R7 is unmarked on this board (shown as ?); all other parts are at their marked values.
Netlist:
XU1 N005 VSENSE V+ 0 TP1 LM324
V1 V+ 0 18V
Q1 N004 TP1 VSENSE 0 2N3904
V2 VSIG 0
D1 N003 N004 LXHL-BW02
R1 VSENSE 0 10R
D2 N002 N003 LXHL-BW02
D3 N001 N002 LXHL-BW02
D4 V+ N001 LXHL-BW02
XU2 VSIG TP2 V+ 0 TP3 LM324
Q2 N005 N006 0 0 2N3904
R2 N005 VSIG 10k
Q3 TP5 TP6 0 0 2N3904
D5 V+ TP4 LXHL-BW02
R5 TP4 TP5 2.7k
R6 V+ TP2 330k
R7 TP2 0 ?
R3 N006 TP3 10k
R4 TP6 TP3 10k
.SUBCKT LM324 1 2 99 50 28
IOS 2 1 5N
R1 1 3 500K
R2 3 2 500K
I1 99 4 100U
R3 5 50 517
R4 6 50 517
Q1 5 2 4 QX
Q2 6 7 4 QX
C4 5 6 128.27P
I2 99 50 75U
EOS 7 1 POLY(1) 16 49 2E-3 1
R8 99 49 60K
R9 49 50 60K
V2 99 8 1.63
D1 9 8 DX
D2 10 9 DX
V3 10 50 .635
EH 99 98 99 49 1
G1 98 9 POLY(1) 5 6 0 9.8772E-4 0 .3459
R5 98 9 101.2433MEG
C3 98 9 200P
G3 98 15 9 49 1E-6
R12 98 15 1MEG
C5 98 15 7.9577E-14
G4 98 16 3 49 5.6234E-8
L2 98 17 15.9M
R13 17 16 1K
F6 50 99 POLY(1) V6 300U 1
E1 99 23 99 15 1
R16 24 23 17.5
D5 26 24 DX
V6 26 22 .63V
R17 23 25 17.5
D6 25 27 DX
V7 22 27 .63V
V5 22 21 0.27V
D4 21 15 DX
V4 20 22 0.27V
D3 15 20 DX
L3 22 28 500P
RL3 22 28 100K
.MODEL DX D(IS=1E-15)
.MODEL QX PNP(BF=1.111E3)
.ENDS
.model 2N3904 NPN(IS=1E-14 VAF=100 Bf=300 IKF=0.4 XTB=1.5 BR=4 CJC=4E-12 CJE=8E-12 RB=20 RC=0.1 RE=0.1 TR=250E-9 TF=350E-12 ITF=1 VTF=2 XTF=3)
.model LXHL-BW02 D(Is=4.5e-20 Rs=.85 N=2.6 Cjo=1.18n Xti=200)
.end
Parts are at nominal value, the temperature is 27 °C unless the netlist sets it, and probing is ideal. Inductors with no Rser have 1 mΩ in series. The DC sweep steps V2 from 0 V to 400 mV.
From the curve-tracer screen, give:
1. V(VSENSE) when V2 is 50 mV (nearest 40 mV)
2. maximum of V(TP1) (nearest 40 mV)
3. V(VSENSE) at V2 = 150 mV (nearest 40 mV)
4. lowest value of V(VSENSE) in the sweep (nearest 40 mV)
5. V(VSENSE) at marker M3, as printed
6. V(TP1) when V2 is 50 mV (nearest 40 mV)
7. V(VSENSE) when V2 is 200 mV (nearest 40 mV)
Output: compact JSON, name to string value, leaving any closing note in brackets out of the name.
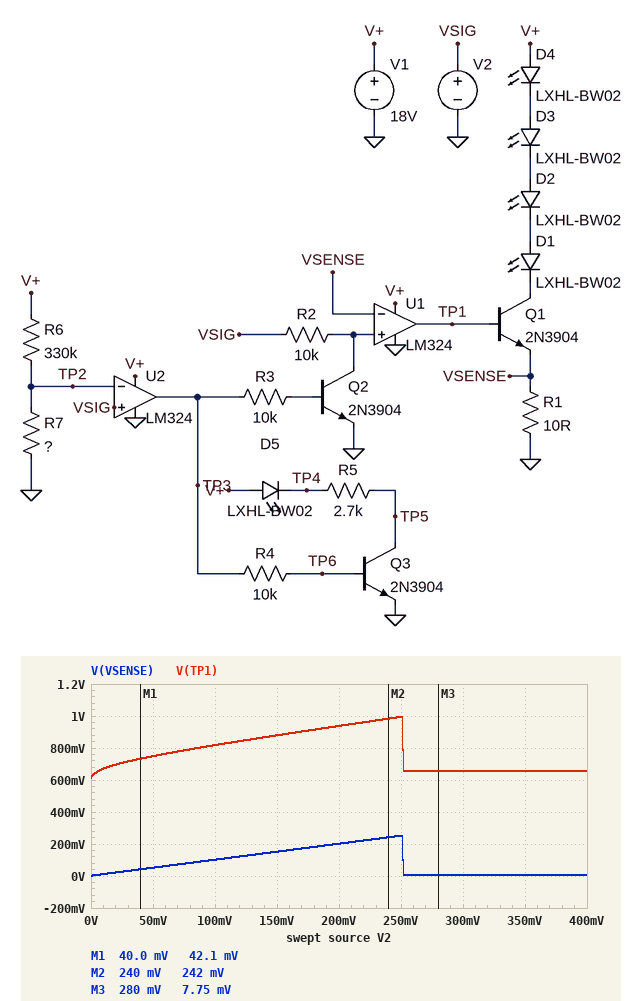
{"V(VSENSE) when V2 is 50 mV": "40 mV", "maximum of V(TP1)": "1.00 V", "V(VSENSE) at V2 = 150 mV": "160 mV", "lowest value of V(VSENSE) in the sweep": "0 V", "V(VSENSE) at marker M3, as printed": "7.75 mV", "V(TP1) when V2 is 50 mV": "760 mV", "V(VSENSE) when V2 is 200 mV": "200 mV"}
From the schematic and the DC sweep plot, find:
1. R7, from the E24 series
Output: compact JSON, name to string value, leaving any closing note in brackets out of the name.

{"R7, from the E24 series": "4.7 kΩ"}
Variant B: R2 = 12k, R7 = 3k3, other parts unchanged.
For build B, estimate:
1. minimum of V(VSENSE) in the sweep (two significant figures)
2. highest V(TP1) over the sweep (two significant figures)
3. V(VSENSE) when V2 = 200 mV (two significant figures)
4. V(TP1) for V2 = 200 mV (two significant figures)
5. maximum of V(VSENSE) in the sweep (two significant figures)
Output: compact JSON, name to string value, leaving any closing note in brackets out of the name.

{"minimum of V(VSENSE) in the sweep": "2.2 mV", "highest V(TP1) over the sweep": "910 mV", "V(VSENSE) when V2 = 200 mV": "7.7 mV", "V(TP1) for V2 = 200 mV": "650 mV", "maximum of V(VSENSE) in the sweep": "180 mV"}
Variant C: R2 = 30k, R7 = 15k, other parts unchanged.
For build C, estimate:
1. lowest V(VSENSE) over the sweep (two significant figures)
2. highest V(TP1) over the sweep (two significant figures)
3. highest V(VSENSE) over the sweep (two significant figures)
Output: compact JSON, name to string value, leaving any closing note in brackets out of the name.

{"lowest V(VSENSE) over the sweep": "3.1 mV", "highest V(TP1) over the sweep": "1.2 V", "highest V(VSENSE) over the sweep": "400 mV"}
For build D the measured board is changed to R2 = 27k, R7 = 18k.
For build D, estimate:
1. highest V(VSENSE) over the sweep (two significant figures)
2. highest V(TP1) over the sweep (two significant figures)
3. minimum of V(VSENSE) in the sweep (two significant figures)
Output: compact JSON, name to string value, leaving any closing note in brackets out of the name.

{"highest V(VSENSE) over the sweep": "400 mV", "highest V(TP1) over the sweep": "1.2 V", "minimum of V(VSENSE) in the sweep": "3.0 mV"}
